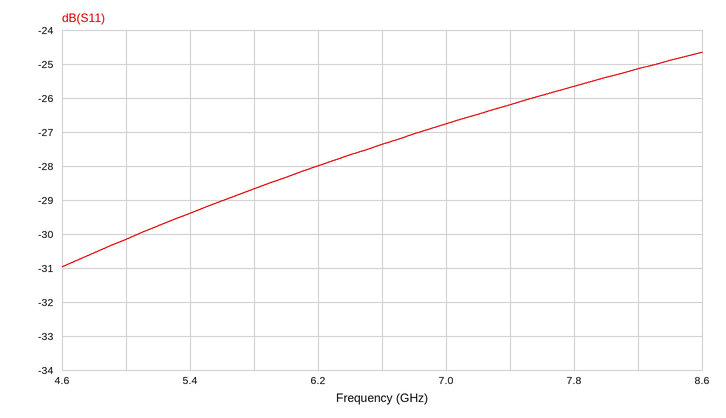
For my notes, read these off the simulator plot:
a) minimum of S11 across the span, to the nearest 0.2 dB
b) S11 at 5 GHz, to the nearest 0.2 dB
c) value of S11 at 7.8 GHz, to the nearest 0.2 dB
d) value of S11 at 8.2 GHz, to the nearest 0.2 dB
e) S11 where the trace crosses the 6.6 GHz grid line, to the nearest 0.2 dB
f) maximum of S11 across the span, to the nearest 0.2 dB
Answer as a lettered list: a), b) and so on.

a) -31.0 dB
b) -30.2 dB
c) -25.6 dB
d) -25.2 dB
e) -27.4 dB
f) -24.6 dB
